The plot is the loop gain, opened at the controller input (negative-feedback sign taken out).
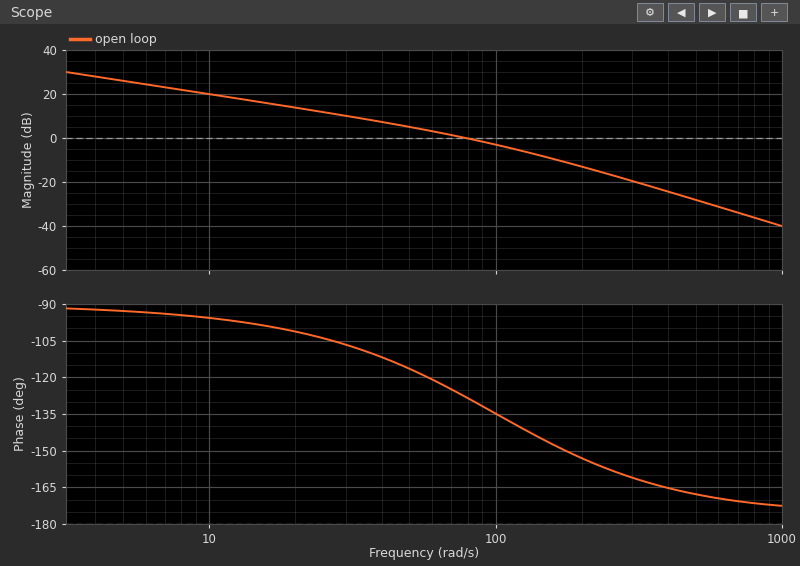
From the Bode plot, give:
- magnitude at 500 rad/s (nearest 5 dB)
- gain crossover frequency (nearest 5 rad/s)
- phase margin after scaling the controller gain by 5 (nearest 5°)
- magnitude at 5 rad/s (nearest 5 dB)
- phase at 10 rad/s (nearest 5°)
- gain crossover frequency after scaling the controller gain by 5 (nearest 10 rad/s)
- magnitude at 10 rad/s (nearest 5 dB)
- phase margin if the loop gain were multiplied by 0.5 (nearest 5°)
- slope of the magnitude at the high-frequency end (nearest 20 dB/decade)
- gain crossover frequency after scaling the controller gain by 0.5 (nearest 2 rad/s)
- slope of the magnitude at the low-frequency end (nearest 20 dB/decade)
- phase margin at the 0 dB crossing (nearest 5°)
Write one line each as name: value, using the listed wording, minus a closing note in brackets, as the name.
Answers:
magnitude at 500 rad/s: -30 dB
gain crossover frequency: 80 rad/s
phase margin after scaling the controller gain by 5: 25°
magnitude at 5 rad/s: 25 dB
phase at 10 rad/s: -95°
gain crossover frequency after scaling the controller gain by 5: 210 rad/s
magnitude at 10 rad/s: 20 dB
phase margin if the loop gain were multiplied by 0.5: 65°
slope of the magnitude at the high-frequency end: -40 dB/decade
gain crossover frequency after scaling the controller gain by 0.5: 46 rad/s
slope of the magnitude at the low-frequency end: -20 dB/decade
phase margin at the 0 dB crossing: 50°
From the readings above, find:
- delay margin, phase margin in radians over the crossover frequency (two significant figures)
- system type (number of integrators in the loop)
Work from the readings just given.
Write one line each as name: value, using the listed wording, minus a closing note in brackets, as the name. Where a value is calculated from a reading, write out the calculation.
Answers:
delay margin, phase margin in radians over the crossover frequency: 50 × π / 180 / 80 = 0.011 s
system type: 1
